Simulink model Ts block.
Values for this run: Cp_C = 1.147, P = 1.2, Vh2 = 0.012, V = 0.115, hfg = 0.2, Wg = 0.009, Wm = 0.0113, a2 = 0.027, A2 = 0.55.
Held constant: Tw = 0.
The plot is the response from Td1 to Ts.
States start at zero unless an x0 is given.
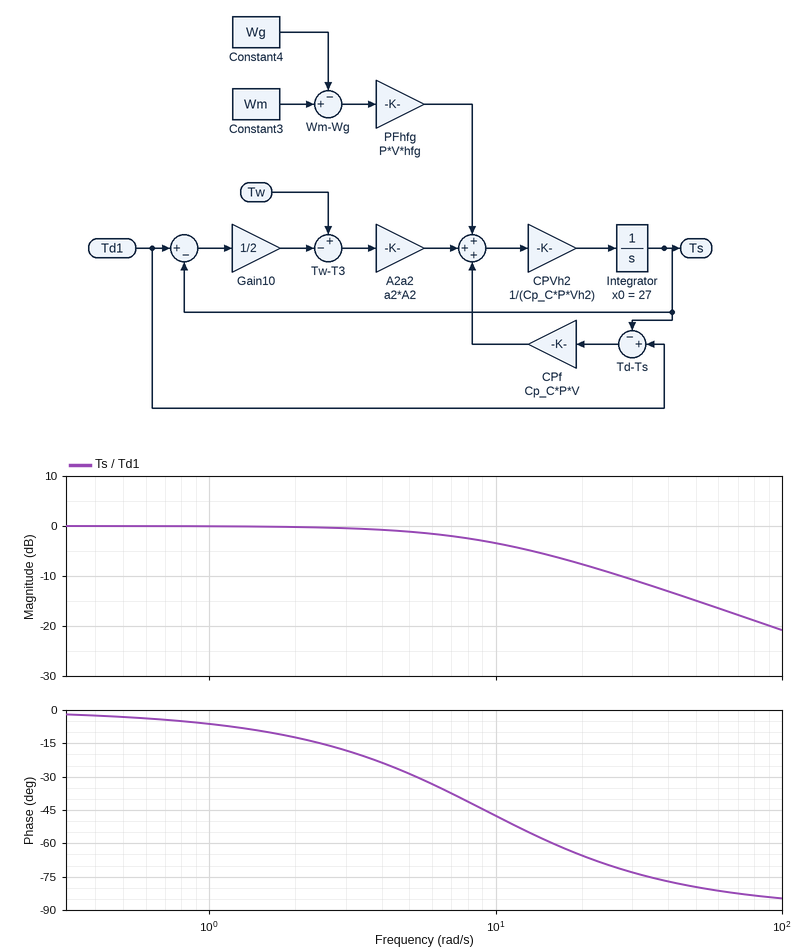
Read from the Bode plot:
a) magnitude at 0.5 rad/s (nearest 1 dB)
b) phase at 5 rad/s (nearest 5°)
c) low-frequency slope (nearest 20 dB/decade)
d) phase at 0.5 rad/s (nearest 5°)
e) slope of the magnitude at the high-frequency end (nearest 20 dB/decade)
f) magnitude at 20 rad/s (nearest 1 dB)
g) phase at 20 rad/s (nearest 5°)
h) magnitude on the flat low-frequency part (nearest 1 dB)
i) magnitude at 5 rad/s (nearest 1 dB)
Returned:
0 dB
-30°
0 dB/decade
-5°
-20 dB/decade
-8 dB
-65°
0 dB
-1 dB
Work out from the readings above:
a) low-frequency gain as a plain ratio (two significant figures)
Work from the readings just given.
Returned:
1.0
